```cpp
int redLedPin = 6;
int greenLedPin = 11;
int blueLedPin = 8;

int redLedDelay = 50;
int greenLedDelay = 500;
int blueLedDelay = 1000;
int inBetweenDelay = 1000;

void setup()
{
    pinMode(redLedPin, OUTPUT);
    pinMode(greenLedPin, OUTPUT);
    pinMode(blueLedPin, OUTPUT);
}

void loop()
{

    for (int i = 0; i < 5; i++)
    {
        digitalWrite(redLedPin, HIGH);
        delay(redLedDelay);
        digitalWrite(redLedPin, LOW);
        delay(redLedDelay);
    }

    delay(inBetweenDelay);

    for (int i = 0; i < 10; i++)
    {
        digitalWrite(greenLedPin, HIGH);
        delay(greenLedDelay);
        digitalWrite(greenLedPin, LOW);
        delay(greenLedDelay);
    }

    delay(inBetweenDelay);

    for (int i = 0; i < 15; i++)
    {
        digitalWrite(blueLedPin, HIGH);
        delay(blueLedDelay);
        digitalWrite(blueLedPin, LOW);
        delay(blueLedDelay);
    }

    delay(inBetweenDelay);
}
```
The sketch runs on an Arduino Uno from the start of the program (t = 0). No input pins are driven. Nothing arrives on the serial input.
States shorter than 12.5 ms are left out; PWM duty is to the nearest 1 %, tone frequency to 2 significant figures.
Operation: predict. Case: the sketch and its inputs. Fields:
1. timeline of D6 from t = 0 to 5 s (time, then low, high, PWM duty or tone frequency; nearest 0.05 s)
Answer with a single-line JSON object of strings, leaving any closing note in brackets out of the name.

{"timeline of D6 from t = 0 to 5 s": "0 s high; 0.05 s low; 0.1 s high; 0.15 s low; 0.2 s high; 0.25 s low; 0.3 s high; 0.35 s low; 0.4 s high; 0.45 s low"}
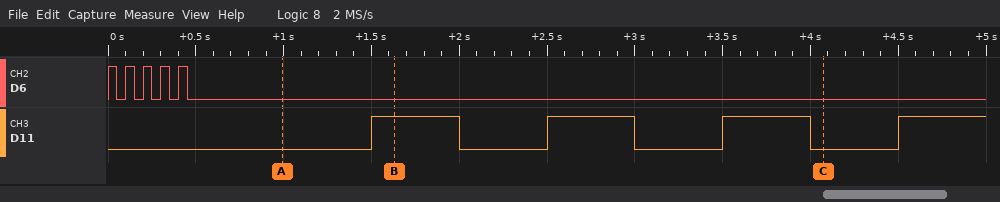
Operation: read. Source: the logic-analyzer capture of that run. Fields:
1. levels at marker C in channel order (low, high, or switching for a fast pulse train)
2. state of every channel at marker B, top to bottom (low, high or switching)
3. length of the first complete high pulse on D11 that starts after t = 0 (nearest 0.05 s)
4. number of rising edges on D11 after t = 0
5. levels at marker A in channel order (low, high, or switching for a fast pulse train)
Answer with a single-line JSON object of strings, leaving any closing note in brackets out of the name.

{"levels at marker C in channel order": "D6 low, D11 low", "state of every channel at marker B, top to bottom": "D6 low, D11 high", "length of the first complete high pulse on D11 that starts after t = 0": "0.50 s", "number of rising edges on D11 after t = 0": "4", "levels at marker A in channel order": "D6 low, D11 low"}
